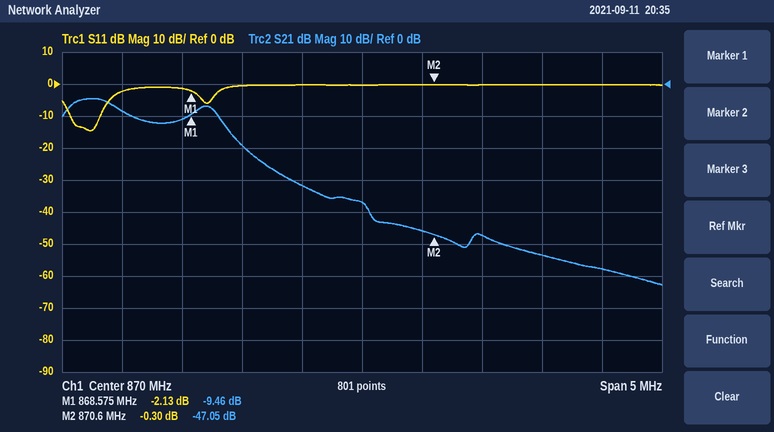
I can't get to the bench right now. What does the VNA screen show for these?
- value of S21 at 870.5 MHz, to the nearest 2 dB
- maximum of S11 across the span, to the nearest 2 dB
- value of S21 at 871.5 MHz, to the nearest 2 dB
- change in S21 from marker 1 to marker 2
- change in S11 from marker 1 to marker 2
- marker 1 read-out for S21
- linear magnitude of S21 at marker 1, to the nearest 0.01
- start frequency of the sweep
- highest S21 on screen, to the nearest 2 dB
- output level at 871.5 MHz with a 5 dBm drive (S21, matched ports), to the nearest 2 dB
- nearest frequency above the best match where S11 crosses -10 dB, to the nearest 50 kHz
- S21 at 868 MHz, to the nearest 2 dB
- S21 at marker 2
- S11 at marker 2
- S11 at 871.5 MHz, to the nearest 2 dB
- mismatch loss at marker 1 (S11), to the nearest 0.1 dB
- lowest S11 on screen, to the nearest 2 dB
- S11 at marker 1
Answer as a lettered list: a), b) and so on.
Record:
a) -46 dB
b) 0 dB
c) -54 dB
d) -37.59 dB
e) 1.83 dB
f) -9.46 dB
g) 0.34
h) 867.5 MHz
i) -4 dB
j) -48 dBm
k) 867.80 MHz
l) -8 dB
m) -47.05 dB
n) -0.30 dB
o) 0 dB
p) 4.1 dB
q) -14 dB
r) -2.13 dB
